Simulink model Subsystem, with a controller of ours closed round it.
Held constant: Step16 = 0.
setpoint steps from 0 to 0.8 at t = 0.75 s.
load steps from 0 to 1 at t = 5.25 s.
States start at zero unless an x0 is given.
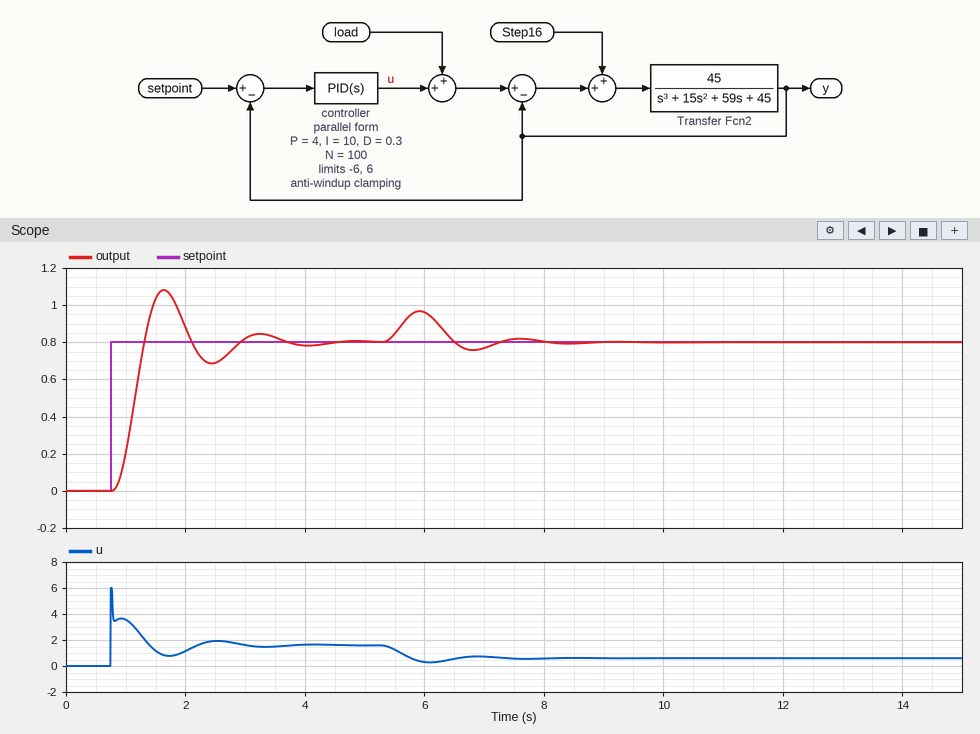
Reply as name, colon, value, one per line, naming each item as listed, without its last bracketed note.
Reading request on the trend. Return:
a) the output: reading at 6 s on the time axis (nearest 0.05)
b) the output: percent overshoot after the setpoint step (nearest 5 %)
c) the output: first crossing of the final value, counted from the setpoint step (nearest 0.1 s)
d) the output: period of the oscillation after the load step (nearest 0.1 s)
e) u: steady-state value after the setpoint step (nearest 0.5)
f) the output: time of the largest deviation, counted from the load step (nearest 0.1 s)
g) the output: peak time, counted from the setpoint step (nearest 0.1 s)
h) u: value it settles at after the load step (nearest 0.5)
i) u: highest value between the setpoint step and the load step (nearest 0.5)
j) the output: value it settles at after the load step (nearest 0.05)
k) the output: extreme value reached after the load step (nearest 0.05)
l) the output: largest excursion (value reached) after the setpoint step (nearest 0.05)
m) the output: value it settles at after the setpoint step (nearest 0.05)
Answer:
the output: reading at 6 s on the time axis: 0.95
the output: percent overshoot after the setpoint step: 35 %
the output: first crossing of the final value, counted from the setpoint step: 0.6 s
the output: period of the oscillation after the load step: 1.7 s
u: steady-state value after the setpoint step: 1.5
the output: time of the largest deviation, counted from the load step: 0.7 s
the output: peak time, counted from the setpoint step: 0.9 s
u: value it settles at after the load step: 0.5
u: highest value between the setpoint step and the load step: 6.0
the output: value it settles at after the load step: 0.80
the output: extreme value reached after the load step: 0.95
the output: largest excursion (value reached) after the setpoint step: 1.10
the output: value it settles at after the setpoint step: 0.80
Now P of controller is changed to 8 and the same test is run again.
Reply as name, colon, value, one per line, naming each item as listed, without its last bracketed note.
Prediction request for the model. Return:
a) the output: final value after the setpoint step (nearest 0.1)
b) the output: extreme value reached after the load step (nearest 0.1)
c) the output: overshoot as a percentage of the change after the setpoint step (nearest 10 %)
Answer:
the output: final value after the setpoint step: 0.8
the output: extreme value reached after the load step: 0.9
the output: overshoot as a percentage of the change after the setpoint step: 30 %
